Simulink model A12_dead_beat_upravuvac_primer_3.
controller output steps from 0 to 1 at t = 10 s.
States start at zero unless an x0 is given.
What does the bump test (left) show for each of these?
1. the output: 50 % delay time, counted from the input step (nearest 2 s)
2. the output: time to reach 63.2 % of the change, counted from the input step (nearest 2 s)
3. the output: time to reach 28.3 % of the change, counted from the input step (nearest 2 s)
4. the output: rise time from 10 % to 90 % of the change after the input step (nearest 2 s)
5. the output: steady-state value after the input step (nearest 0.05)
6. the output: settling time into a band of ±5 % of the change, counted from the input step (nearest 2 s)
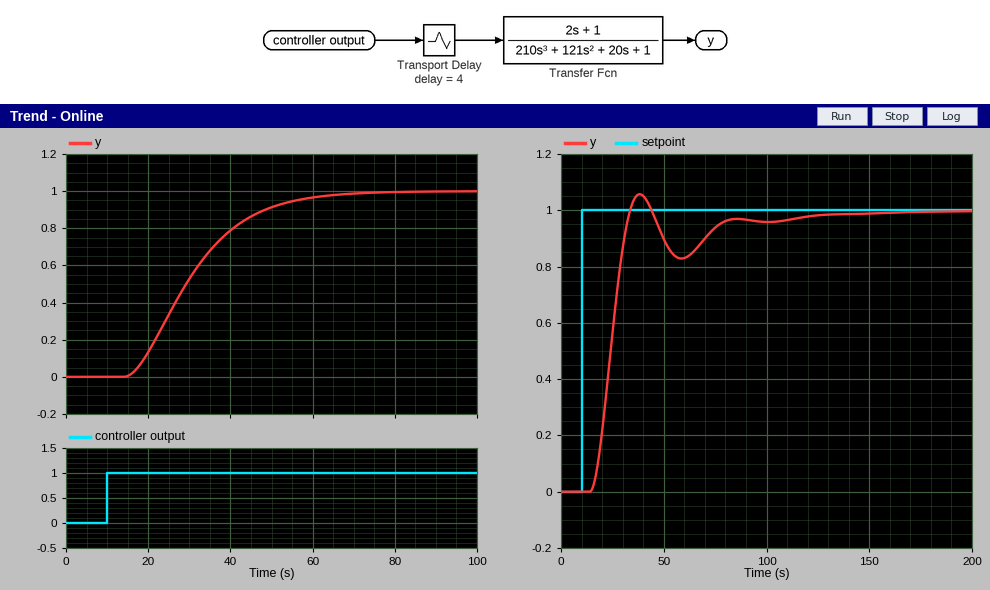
20 s
24 s
14 s
30 s
1.00
46 s
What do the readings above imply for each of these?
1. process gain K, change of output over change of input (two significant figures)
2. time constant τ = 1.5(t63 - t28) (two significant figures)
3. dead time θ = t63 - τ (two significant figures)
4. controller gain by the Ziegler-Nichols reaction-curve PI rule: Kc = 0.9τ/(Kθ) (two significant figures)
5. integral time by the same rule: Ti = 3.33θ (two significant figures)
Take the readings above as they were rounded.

1.0
15 s
9.0 s
1.5
30 s
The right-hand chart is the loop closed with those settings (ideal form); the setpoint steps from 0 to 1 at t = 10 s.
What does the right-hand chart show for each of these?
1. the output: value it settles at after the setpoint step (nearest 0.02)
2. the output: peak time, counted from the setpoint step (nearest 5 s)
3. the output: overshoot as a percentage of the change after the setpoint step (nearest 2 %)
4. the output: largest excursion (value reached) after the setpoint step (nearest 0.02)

1.00
30 s
6 %
1.06
